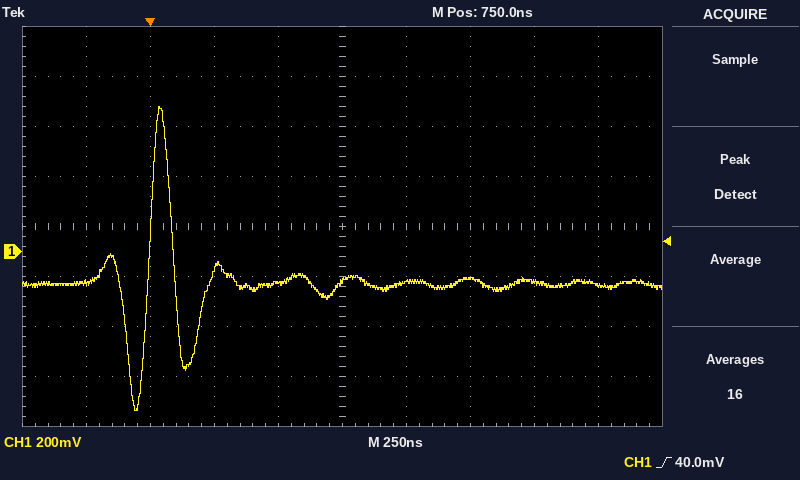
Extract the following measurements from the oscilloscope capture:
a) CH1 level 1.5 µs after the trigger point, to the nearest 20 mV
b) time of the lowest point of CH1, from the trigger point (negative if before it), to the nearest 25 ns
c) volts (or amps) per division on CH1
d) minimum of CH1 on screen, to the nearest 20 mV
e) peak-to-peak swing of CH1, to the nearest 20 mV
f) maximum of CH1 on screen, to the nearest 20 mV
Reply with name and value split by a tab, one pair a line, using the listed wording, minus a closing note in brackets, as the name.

CH1 level 1.5 µs after the trigger point, to the nearest 20 mV	-120 mV
time of the lowest point of CH1, from the trigger point (negative if before it), to the nearest 25 ns	-50 ns
volts (or amps) per division on CH1	200 mV
minimum of CH1 on screen, to the nearest 20 mV	-640 mV
peak-to-peak swing of CH1, to the nearest 20 mV	1.22 V
maximum of CH1 on screen, to the nearest 20 mV	580 mV
